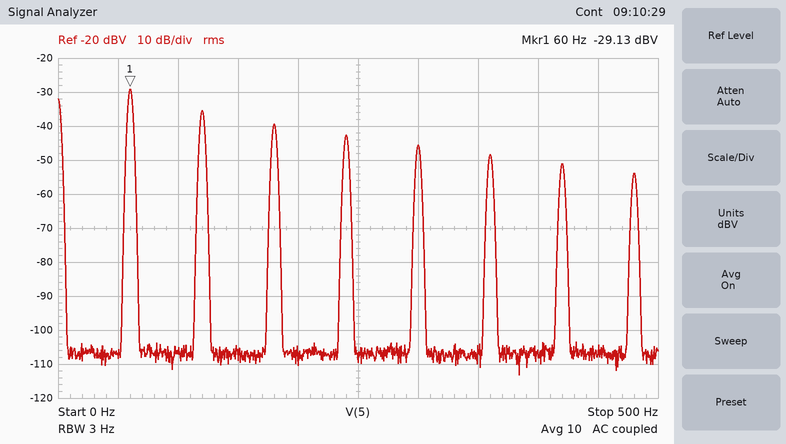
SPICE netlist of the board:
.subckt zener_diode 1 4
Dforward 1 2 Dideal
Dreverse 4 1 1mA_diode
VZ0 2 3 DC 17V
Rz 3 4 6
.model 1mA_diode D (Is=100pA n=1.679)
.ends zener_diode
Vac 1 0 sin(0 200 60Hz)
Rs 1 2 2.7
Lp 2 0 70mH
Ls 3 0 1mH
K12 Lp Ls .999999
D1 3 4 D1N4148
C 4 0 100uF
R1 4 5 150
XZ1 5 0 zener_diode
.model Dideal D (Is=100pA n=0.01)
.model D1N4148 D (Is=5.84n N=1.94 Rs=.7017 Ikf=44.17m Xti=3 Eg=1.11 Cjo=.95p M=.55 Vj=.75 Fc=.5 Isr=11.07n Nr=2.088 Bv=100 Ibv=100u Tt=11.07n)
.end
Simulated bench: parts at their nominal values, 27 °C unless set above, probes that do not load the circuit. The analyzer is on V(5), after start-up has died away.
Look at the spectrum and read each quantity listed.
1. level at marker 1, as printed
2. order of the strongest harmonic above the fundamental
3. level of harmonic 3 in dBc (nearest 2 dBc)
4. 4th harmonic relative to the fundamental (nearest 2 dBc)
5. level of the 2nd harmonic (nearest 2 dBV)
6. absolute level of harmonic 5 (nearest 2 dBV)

-29.13 dBV
2
-10 dBc
-14 dBc
-36 dBV
-46 dBV
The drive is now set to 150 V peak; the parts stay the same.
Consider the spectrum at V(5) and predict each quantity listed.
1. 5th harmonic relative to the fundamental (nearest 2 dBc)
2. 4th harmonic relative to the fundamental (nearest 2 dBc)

-14 dBc
-12 dBc
